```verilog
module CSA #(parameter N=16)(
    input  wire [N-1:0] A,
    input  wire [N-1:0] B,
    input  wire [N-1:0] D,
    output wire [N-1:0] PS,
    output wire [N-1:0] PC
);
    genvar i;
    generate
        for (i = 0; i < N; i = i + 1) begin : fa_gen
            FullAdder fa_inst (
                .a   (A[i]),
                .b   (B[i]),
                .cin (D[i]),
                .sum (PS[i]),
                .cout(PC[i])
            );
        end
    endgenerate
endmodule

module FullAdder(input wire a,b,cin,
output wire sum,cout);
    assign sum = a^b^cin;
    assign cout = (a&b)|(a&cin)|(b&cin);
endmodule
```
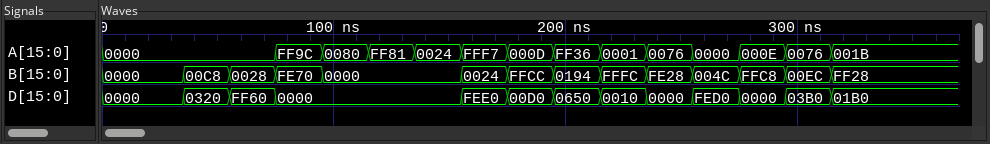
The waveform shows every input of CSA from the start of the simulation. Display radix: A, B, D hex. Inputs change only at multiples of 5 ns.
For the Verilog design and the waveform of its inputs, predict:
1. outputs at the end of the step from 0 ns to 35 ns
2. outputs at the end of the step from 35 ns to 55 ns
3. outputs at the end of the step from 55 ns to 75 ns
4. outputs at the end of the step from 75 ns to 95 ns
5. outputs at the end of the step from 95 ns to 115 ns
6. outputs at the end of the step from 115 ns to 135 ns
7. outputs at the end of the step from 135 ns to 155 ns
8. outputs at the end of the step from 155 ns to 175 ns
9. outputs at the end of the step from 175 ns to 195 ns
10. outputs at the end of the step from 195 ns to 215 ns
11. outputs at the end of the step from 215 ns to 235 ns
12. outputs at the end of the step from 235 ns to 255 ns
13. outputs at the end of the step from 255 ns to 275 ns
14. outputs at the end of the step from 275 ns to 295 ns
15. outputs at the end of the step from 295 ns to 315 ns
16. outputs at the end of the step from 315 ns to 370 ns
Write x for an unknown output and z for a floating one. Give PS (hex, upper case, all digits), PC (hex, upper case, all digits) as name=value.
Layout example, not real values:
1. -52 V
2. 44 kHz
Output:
1. PS=0000, PC=0000
2. PS=03E8, PC=0000
3. PS=FF48, PC=0020
4. PS=01EC, PC=FE10
5. PS=0080, PC=0000
6. PS=FF81, PC=0000
7. PS=0024, PC=0000
8. PS=0133, PC=FEE4
9. PS=FF11, PC=00CC
10. PS=F8F2, PC=0714
11. PS=FFED, PC=0010
12. PS=FE5E, PC=0020
13. PS=FE9C, PC=0040
14. PS=FFC6, PC=0008
15. PS=032A, PC=00F4
16. PS=FE83, PC=0138
